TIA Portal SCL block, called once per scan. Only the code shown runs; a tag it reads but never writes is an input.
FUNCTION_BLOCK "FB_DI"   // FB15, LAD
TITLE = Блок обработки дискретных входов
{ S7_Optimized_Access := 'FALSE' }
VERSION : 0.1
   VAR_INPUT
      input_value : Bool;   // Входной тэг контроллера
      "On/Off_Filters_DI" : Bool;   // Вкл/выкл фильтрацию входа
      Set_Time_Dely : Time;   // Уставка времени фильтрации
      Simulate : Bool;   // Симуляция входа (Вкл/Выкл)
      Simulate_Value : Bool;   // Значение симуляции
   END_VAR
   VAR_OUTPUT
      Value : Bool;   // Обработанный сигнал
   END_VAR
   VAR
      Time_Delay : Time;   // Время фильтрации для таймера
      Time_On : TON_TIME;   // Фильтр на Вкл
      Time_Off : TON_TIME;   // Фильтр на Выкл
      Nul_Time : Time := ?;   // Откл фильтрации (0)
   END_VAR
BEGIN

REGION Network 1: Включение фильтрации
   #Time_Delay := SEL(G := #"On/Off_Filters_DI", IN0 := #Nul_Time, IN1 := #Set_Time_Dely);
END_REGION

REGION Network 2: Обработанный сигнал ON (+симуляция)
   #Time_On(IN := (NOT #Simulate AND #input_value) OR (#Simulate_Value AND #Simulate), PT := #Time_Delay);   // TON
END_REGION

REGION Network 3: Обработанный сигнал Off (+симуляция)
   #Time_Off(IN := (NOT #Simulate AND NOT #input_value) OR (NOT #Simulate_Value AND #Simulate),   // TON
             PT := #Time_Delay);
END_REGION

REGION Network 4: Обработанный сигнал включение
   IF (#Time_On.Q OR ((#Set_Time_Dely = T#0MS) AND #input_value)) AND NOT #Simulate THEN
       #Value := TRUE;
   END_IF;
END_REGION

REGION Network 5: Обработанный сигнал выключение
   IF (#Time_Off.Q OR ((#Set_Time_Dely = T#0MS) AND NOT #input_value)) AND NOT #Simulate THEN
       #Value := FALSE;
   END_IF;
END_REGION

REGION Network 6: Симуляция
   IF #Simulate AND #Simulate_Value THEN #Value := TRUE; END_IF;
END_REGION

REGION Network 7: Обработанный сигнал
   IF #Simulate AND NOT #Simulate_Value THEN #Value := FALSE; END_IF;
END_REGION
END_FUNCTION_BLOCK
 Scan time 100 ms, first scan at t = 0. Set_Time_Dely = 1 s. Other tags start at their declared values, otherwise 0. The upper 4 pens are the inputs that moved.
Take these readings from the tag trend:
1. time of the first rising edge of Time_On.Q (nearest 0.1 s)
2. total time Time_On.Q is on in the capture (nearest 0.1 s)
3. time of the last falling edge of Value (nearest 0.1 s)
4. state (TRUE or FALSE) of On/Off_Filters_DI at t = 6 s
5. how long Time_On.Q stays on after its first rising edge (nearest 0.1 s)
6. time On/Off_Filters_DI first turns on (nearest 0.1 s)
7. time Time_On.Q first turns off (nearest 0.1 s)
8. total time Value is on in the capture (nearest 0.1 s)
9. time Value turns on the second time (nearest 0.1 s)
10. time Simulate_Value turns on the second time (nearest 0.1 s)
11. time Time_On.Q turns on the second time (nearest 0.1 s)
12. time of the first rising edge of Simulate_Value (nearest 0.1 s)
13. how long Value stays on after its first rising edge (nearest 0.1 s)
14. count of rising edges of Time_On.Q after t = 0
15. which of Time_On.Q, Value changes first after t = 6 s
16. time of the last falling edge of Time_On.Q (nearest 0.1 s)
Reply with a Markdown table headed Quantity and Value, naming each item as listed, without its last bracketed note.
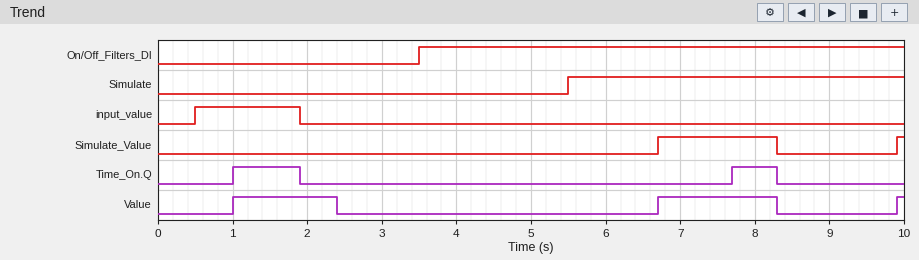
| Quantity | Value |
|---|---|
| time of the first rising edge of Time_On.Q | 1.0 s |
| total time Time_On.Q is on in the capture | 1.5 s |
| time of the last falling edge of Value | 8.3 s |
| state (TRUE or FALSE) of On/Off_Filters_DI at t = 6 s | TRUE |
| how long Time_On.Q stays on after its first rising edge | 0.9 s |
| time On/Off_Filters_DI first turns on | 3.5 s |
| time Time_On.Q first turns off | 1.9 s |
| total time Value is on in the capture | 3.1 s |
| time Value turns on the second time | 6.7 s |
| time Simulate_Value turns on the second time | 9.9 s |
| time Time_On.Q turns on the second time | 7.7 s |
| time of the first rising edge of Simulate_Value | 6.7 s |
| how long Value stays on after its first rising edge | 1.4 s |
| count of rising edges of Time_On.Q after t = 0 | 2 |
| which of Time_On.Q, Value changes first after t = 6 s | Value |
| time of the last falling edge of Time_On.Q | 8.3 s |
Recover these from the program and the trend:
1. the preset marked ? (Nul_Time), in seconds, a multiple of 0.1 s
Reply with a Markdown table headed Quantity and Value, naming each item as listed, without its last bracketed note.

| Quantity | Value |
|---|---|
| the preset marked ? (Nul_Time), in seconds, a multiple of 0.1 s | 0.5 s |
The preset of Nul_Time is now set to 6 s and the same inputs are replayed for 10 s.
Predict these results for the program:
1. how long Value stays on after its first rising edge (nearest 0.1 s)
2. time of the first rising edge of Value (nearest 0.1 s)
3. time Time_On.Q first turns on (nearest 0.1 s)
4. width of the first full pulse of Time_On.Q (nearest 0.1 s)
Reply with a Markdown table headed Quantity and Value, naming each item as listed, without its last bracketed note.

| Quantity | Value |
|---|---|
| how long Value stays on after its first rising edge | 1.6 s |
| time of the first rising edge of Value | 6.7 s |
| time Time_On.Q first turns on | 7.7 s |
| width of the first full pulse of Time_On.Q | 0.6 s |
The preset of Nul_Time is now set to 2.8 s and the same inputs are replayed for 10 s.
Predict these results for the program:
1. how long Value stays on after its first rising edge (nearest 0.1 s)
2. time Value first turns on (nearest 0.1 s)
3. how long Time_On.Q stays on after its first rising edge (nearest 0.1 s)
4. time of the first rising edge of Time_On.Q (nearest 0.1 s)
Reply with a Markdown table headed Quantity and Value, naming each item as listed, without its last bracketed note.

| Quantity | Value |
|---|---|
| how long Value stays on after its first rising edge | 1.6 s |
| time Value first turns on | 6.7 s |
| how long Time_On.Q stays on after its first rising edge | 0.6 s |
| time of the first rising edge of Time_On.Q | 7.7 s |
